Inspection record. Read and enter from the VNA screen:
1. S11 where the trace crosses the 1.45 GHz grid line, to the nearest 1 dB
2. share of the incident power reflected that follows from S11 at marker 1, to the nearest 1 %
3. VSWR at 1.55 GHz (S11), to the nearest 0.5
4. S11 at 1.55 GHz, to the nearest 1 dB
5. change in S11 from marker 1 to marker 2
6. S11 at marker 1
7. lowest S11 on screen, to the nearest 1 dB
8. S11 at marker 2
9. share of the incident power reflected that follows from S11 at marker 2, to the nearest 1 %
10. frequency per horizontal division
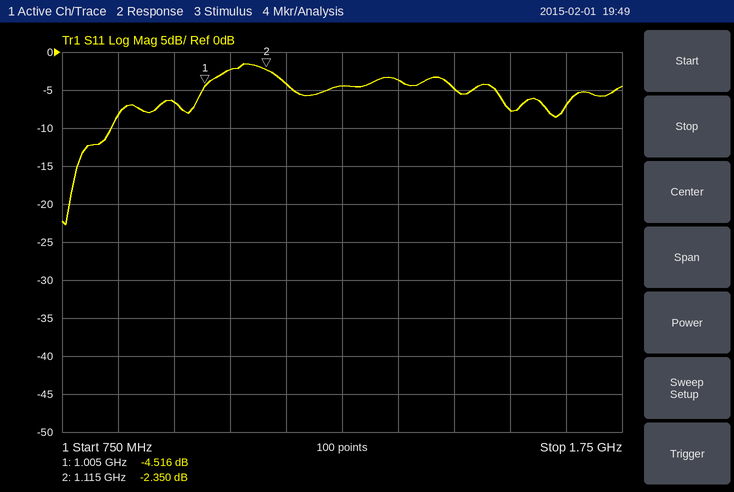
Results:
-5 dB
35 %
2.5
-8 dB
2.166 dB
-4.516 dB
-23 dB
-2.350 dB
58 %
100 MHz
